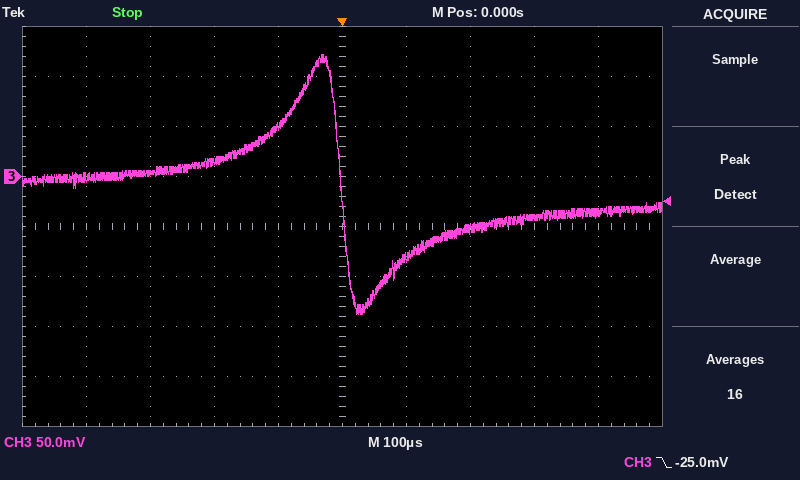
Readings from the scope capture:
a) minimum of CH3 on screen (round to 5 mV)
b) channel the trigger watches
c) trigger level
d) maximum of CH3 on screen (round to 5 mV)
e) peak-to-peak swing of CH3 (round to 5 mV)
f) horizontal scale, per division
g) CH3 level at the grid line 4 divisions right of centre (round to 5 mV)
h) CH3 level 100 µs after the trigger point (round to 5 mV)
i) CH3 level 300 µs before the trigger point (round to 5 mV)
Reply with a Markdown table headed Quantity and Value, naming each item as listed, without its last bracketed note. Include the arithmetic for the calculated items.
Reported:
| Quantity | Value |
|---|---|
| minimum of CH3 on screen | -140 mV |
| channel the trigger watches | CH3 |
| trigger level | -25.0 mV |
| maximum of CH3 on screen | 120 mV |
| peak-to-peak swing of CH3 | 120 mV − (-140 mV) = 260 mV |
| horizontal scale, per division | 100 µs |
| CH3 level at the grid line 4 divisions right of centre | -35 mV |
| CH3 level 100 µs after the trigger point | -80 mV |
| CH3 level 300 µs before the trigger point | 5 mV |
